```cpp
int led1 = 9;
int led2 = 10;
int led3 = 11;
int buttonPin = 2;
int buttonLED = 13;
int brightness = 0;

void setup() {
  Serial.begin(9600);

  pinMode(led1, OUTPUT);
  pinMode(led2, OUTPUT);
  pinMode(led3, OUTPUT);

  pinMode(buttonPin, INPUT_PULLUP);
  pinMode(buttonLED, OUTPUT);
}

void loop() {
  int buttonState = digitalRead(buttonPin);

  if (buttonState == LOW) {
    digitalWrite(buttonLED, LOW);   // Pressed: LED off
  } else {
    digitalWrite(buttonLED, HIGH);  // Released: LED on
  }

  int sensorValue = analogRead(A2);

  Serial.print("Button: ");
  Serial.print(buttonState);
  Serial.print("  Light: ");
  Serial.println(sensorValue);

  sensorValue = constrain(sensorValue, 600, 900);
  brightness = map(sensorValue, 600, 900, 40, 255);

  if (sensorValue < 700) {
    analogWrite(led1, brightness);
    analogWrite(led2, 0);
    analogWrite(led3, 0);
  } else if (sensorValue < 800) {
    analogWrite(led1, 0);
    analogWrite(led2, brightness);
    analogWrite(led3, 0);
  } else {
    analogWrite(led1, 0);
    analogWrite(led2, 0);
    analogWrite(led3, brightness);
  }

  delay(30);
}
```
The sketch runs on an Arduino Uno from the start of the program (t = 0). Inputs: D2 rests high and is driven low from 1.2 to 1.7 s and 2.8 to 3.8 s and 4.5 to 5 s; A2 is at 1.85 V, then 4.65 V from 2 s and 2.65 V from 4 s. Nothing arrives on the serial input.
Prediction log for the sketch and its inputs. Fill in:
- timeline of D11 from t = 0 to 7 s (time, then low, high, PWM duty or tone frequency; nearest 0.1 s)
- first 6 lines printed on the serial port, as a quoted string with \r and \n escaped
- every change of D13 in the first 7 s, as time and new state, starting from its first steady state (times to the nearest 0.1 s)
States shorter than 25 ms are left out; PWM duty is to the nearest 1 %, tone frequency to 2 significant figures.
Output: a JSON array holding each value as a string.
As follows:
["0 s low; 2 s high; 4 s low", "\"Button: 1  Light: 378\\r\\nButton: 1  Light: 378\\r\\nButton: 1  Light: 378\\r\\nButton: 1  Light: 378\\r\\nButton: 1  Light: 378\\r\\nButton: 1  Light: 378\\r\\n\"", "0 s high; 1.2 s low; 1.7 s high; 2.8 s low; 3.8 s high; 4.5 s low; 5 s high"]
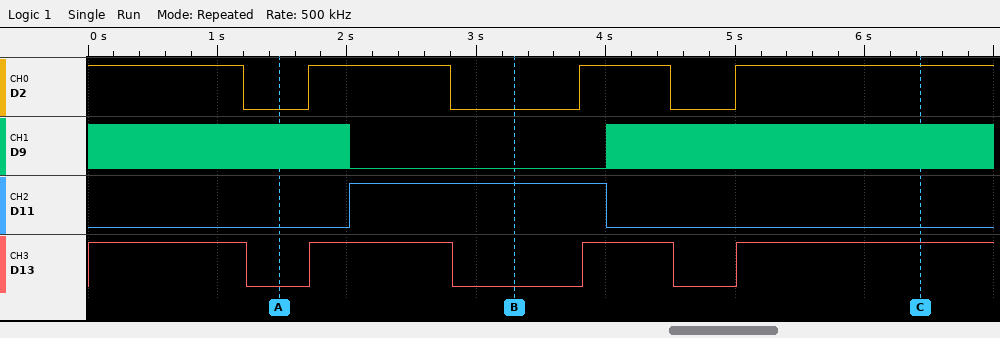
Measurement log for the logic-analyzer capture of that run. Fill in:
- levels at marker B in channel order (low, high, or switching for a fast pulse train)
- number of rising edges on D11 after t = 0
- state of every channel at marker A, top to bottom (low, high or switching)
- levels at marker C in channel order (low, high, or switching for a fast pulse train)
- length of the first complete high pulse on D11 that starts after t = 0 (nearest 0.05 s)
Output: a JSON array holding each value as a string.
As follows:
["D2 low, D9 low, D11 high, D13 low", "1", "D2 low, D9 switching, D11 low, D13 low", "D2 high, D9 switching, D11 low, D13 high", "2.00 s"]
